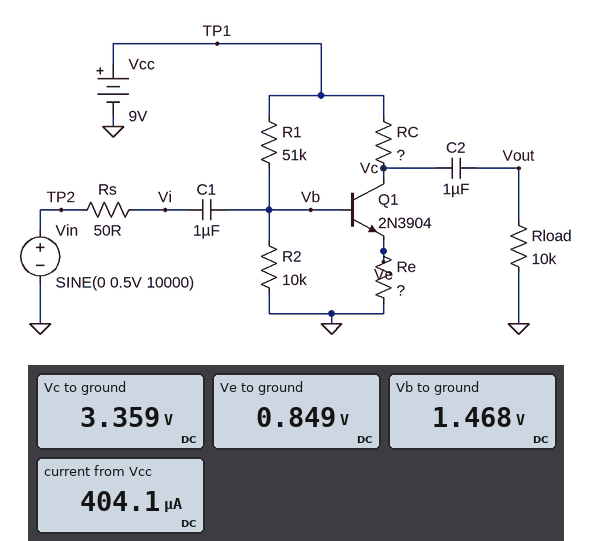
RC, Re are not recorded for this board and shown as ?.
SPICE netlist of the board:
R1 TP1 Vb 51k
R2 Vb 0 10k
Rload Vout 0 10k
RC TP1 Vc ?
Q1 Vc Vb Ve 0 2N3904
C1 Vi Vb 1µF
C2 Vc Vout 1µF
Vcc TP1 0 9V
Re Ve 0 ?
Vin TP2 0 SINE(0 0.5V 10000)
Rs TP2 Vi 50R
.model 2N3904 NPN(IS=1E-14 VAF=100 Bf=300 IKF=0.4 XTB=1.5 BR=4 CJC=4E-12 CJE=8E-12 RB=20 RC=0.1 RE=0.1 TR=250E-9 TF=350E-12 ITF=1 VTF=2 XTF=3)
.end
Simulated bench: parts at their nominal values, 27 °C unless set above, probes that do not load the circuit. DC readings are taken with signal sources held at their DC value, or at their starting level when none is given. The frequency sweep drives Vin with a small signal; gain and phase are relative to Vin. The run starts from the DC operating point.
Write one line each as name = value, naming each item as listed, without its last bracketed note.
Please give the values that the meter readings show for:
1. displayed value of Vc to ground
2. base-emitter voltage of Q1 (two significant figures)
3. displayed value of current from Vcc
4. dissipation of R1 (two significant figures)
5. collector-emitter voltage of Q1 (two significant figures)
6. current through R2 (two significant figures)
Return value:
displayed value of Vc to ground = 3.359 V
base-emitter voltage of Q1 = 620 mV
displayed value of current from Vcc = 404.1 µA
dissipation of R1 = 1.1 mW
collector-emitter voltage of Q1 = 2.5 V
current through R2 = 150 µA
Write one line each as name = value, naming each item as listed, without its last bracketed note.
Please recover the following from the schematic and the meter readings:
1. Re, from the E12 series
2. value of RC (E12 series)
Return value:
Re, from the E12 series = 3.3 kΩ
value of RC = 22 kΩ
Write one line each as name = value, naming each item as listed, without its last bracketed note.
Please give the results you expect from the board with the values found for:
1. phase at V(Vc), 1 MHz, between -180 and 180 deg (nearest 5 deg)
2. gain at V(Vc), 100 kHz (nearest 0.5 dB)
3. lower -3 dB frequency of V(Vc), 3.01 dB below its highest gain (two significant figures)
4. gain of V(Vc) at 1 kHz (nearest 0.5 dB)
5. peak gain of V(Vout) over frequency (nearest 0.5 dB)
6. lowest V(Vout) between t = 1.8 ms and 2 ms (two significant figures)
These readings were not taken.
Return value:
phase at V(Vc), 1 MHz, between -180 and 180 deg = 170 deg
gain at V(Vc), 100 kHz = 6.0 dB
lower -3 dB frequency of V(Vc), 3.01 dB below its highest gain = 7.3 Hz
gain of V(Vc) at 1 kHz = 6.0 dB
peak gain of V(Vout) over frequency = 6.0 dB
lowest V(Vout) between t = 1.8 ms and 2 ms = -1.0 V
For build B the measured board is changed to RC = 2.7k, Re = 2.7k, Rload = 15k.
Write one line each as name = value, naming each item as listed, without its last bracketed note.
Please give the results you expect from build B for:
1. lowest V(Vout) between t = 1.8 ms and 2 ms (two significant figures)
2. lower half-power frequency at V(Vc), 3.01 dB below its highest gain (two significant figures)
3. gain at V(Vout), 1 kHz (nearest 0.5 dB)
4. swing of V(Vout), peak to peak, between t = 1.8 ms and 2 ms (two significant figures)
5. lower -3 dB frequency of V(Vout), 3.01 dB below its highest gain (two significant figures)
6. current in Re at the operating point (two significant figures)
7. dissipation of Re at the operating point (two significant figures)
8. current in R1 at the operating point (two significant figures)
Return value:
lowest V(Vout) between t = 1.8 ms and 2 ms = -410 mV
lower half-power frequency at V(Vc), 3.01 dB below its highest gain = 37 Hz
gain at V(Vout), 1 kHz = -2.0 dB
swing of V(Vout), peak to peak, between t = 1.8 ms and 2 ms = 810 mV
lower -3 dB frequency of V(Vout), 3.01 dB below its highest gain = 43 Hz
current in Re at the operating point = 310 µA
dissipation of Re at the operating point = 260 µW
current in R1 at the operating point = 150 µA
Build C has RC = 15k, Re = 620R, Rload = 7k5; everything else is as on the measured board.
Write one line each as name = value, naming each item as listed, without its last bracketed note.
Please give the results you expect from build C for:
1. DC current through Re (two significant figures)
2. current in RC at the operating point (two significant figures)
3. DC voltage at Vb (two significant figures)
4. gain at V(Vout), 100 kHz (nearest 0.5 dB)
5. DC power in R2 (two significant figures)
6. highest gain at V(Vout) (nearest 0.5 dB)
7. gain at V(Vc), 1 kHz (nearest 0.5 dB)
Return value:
DC current through Re = 620 µA
current in RC at the operating point = 570 µA
DC voltage at Vb = 1.0 V
gain at V(Vout), 100 kHz = -6.5 dB
DC power in R2 = 110 µW
highest gain at V(Vout) = -1.0 dB
gain at V(Vc), 1 kHz = -11.0 dB
